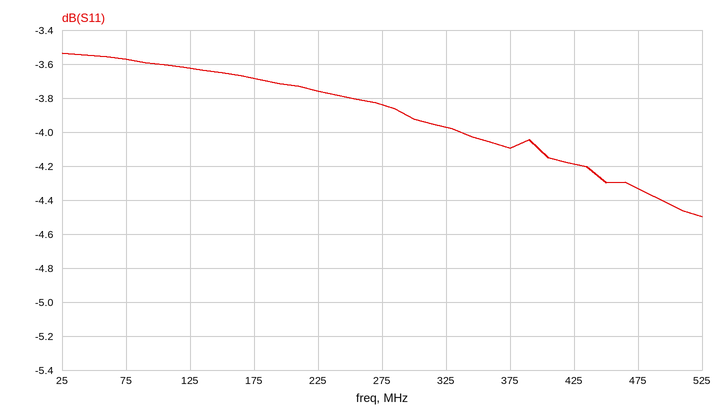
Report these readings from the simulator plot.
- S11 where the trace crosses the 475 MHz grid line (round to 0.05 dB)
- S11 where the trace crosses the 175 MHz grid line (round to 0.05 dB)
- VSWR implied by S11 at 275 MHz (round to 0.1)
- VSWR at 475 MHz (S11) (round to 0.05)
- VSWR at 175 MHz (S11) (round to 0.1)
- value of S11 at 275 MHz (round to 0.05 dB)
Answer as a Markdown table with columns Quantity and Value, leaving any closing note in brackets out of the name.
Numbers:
| Quantity | Value |
|---|---|
| S11 where the trace crosses the 475 MHz grid line | -4.35 dB |
| S11 where the trace crosses the 175 MHz grid line | -3.70 dB |
| VSWR implied by S11 at 275 MHz | 4.6 |
| VSWR at 475 MHz (S11) | 4.10 |
| VSWR at 175 MHz (S11) | 4.8 |
| value of S11 at 275 MHz | -3.85 dB |
